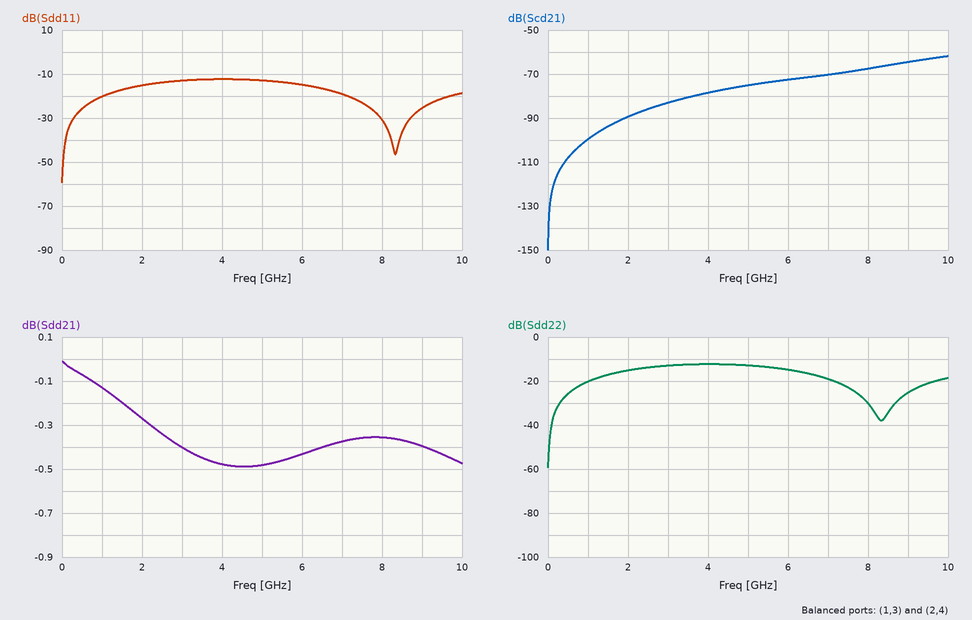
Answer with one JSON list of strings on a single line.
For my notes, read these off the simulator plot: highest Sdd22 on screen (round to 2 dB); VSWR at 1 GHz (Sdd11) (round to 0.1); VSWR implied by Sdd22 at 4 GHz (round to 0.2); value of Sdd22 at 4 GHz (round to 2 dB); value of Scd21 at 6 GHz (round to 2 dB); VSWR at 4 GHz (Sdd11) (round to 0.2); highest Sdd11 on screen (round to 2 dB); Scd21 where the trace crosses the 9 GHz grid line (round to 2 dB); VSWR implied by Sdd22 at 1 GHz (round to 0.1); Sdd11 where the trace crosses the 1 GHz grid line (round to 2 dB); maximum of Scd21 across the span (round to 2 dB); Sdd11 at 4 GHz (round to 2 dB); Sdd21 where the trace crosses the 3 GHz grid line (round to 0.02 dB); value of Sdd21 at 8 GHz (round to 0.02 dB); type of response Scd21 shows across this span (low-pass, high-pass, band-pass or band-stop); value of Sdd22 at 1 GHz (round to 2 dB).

["-12 dB", "1.2", "1.6", "-12 dB", "-72 dB", "1.6", "-12 dB", "-64 dB", "1.2", "-20 dB", "-62 dB", "-12 dB", "-0.40 dB", "-0.36 dB", "high-pass", "-20 dB"]
